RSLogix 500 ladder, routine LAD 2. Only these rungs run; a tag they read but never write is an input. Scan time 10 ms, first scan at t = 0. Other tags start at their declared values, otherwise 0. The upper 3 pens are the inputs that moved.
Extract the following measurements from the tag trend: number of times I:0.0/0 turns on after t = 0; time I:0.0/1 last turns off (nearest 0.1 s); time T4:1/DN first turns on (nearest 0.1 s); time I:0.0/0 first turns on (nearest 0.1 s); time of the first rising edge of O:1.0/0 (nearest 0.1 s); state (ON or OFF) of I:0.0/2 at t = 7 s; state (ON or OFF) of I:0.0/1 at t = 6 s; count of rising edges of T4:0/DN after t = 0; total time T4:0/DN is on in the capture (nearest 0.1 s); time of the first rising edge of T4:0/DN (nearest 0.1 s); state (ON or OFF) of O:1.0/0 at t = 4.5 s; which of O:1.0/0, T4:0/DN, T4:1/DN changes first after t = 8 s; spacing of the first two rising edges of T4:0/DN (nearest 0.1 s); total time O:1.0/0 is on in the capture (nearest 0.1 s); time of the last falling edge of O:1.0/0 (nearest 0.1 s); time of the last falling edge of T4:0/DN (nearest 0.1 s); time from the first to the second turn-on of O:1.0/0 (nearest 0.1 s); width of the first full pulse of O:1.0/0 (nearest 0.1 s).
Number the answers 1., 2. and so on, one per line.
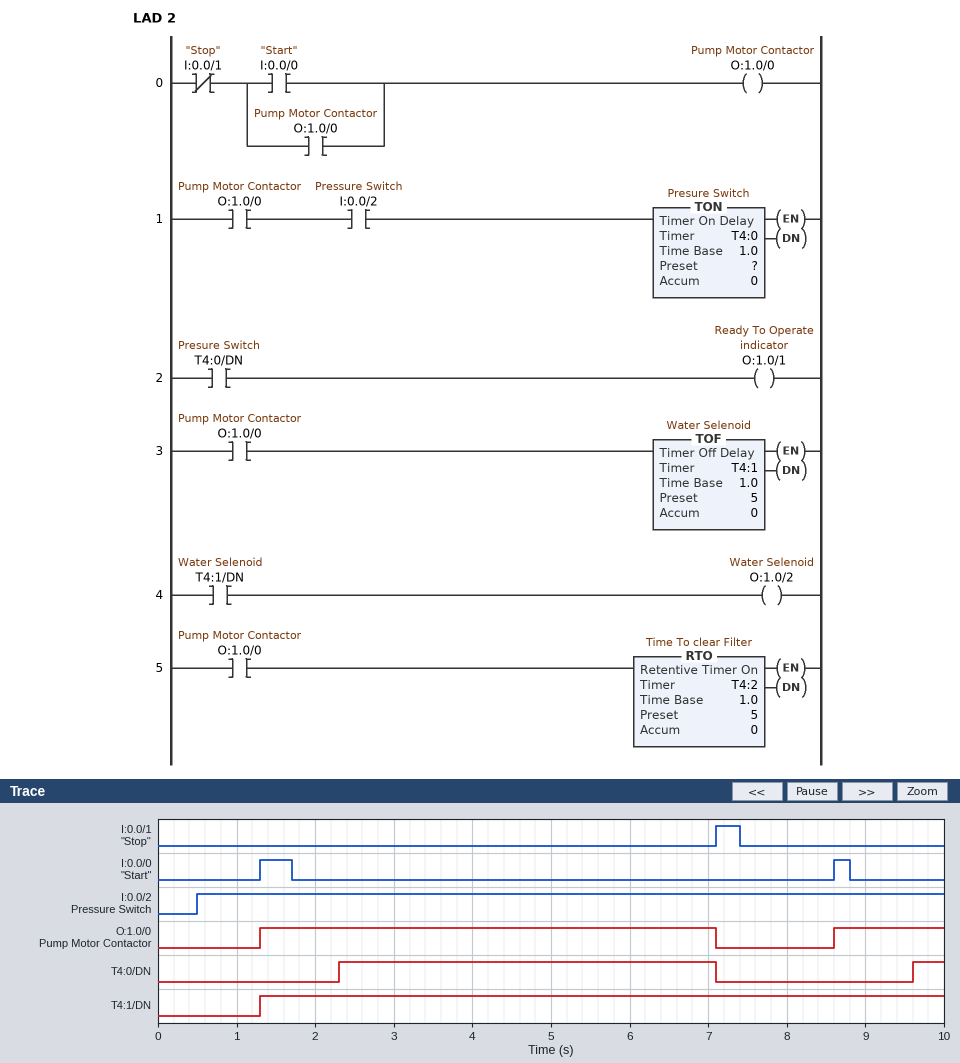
1. 2
2. 7.4 s
3. 1.3 s
4. 1.3 s
5. 1.3 s
6. ON
7. OFF
8. 2
9. 5.2 s
10. 2.3 s
11. ON
12. O:1.0/0
13. 7.3 s
14. 7.2 s
15. 7.1 s
16. 7.1 s
17. 7.3 s
18. 5.8 s
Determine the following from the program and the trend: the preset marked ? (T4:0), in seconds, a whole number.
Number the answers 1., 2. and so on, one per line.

1. 1 s
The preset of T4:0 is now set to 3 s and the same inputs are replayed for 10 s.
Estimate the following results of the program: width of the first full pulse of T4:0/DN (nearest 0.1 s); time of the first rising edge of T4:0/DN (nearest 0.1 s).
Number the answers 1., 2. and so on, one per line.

1. 2.8 s
2. 4.3 s
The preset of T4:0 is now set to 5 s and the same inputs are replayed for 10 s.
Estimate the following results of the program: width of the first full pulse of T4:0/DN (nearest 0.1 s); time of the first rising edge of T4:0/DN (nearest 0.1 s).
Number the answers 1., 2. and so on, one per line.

1. 0.8 s
2. 6.3 s
